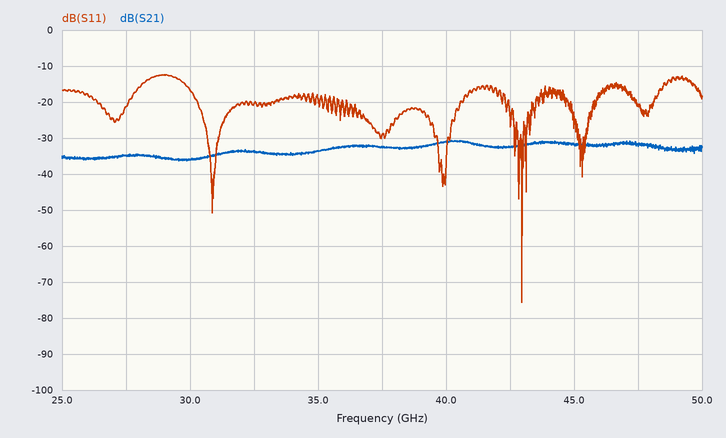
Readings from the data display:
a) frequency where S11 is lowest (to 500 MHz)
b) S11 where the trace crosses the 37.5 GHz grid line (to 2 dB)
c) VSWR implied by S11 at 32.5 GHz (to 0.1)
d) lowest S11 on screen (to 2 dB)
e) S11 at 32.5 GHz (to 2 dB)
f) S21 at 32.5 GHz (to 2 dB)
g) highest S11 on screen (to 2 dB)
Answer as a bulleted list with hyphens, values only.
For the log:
- 43.0 GHz
- -30 dB
- 1.2
- -76 dB
- -20 dB
- -34 dB
- -12 dB
